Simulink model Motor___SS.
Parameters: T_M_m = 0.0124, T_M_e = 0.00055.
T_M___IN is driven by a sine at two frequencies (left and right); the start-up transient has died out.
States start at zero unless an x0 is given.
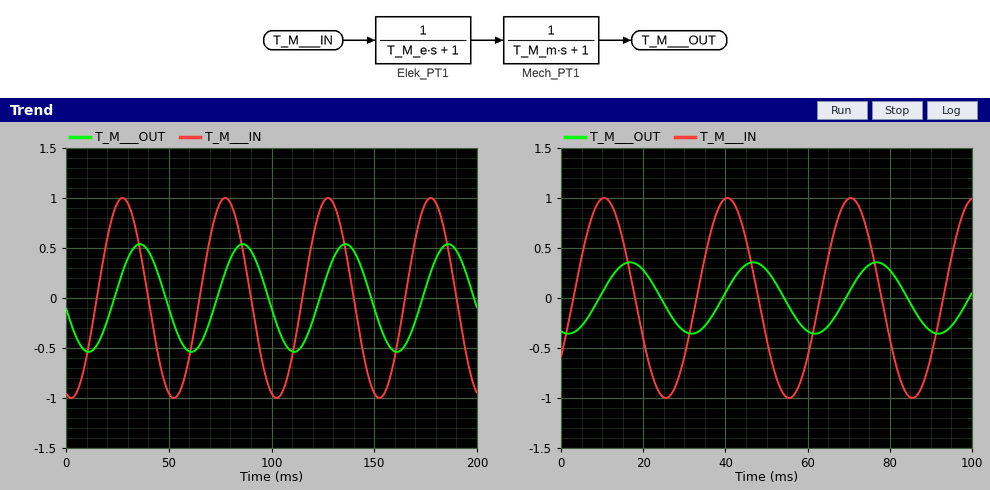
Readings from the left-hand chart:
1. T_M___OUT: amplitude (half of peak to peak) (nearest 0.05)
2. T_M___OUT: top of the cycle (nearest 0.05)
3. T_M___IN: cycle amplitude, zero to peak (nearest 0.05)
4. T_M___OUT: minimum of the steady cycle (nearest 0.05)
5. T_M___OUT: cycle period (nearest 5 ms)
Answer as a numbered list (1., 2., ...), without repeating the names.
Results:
1. 0.55
2. 0.55
3. 1.00
4. -0.55
5. 50 ms
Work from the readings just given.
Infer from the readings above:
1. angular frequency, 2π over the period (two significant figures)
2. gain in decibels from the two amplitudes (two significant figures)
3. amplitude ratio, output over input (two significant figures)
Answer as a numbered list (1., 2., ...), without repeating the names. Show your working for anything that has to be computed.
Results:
1. 2π / 50 = 0.13 rad/ms
2. 20 log10(0.55 / 1) = -5.2 dB
3. 0.55 / 1 = 0.55
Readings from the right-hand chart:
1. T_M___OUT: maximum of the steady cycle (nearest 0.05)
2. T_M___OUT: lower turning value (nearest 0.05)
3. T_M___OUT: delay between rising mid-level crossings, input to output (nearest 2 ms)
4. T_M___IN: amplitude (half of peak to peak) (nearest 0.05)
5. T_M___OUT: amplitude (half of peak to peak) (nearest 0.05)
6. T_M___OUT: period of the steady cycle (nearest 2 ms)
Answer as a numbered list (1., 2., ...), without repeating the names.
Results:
1. 0.35
2. -0.35
3. 6 ms
4. 1.00
5. 0.35
6. 30 ms
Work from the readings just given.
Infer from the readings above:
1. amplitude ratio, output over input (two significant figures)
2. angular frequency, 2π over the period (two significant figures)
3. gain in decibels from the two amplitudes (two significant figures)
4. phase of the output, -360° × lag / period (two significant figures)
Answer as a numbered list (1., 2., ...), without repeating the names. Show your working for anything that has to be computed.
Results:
1. 0.35 / 1 = 0.35
2. 2π / 30 = 0.21 rad/ms
3. 20 log10(0.35 / 1) = -9.1 dB
4. -360 × 6 / 30 = -72°
